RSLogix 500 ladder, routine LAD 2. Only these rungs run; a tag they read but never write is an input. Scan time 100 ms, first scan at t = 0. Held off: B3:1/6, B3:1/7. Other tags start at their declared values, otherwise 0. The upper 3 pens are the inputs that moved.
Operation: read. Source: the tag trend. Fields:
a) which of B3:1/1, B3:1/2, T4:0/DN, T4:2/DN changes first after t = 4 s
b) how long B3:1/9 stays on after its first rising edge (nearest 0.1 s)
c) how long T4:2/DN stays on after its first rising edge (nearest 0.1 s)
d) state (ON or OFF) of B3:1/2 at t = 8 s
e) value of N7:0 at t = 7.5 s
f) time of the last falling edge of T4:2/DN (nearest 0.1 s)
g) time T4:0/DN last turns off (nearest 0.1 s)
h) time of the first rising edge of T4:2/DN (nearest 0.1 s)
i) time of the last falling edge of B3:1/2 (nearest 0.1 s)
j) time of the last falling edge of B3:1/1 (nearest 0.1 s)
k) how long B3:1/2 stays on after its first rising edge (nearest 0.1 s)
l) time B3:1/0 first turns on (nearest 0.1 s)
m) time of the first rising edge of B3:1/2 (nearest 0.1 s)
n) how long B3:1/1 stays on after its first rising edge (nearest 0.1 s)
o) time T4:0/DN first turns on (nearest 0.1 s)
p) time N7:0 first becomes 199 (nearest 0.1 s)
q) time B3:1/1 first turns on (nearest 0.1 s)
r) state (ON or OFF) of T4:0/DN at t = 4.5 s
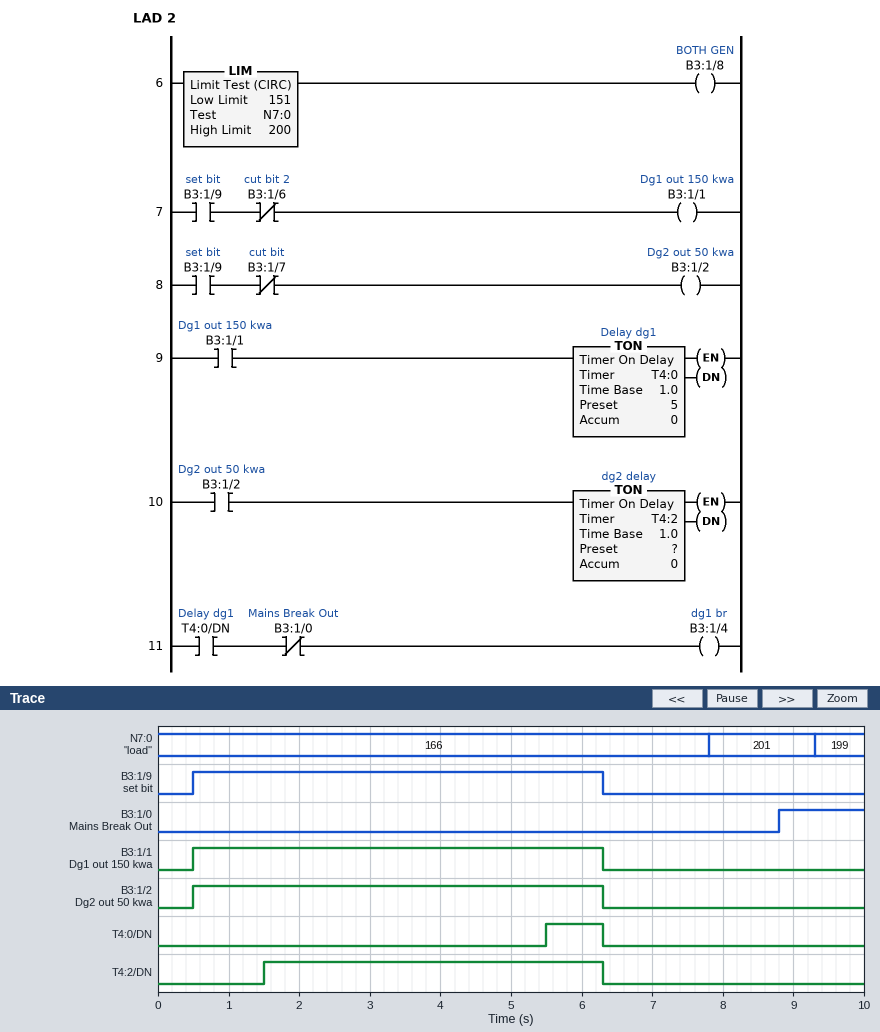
T4:0/DN
5.8 s
4.8 s
OFF
166
6.3 s
6.3 s
1.5 s
6.3 s
6.3 s
5.8 s
8.8 s
0.5 s
5.8 s
5.5 s
9.3 s
0.5 s
OFF
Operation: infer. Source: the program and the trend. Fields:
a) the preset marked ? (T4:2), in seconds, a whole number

1 s
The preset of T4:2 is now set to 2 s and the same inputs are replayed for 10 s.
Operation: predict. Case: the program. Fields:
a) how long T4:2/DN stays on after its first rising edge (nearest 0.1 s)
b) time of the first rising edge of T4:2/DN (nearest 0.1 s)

3.8 s
2.5 s
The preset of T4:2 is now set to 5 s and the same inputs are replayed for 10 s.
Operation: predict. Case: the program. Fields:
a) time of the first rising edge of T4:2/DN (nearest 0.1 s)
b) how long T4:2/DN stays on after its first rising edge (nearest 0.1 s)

5.5 s
0.8 s
